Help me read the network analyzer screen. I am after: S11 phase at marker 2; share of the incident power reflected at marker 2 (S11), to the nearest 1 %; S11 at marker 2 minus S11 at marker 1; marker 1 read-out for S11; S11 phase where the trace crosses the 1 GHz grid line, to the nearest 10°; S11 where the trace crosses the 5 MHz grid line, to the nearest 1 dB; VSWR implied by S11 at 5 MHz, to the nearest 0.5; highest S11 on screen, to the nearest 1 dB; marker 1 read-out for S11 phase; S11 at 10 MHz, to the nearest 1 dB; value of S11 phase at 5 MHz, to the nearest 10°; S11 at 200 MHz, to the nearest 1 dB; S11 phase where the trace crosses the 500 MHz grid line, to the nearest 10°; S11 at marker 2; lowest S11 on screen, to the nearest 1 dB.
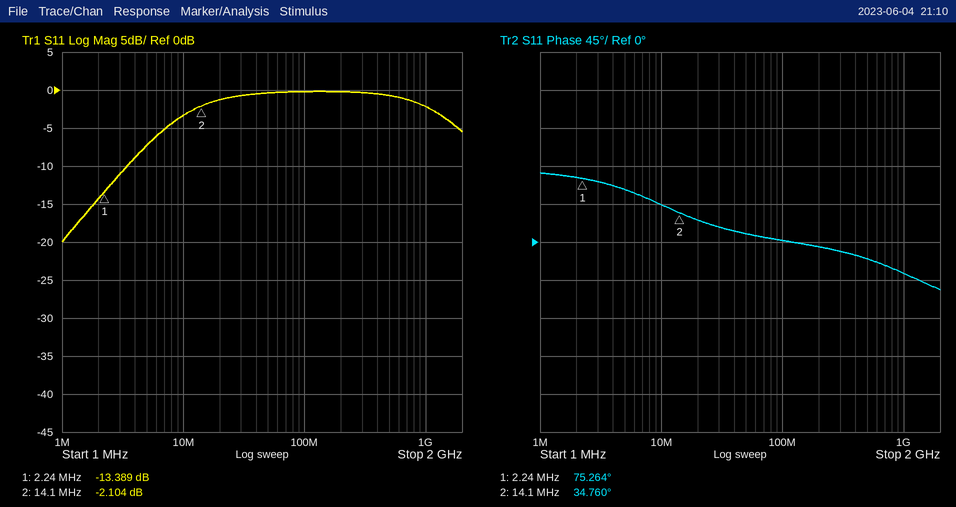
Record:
34.760°
62 %
11.285 dB
-13.389 dB
-40°
-7 dB
2.5
0 dB
75.264°
-3 dB
60°
0 dB
-20°
-2.104 dB
-20 dB
